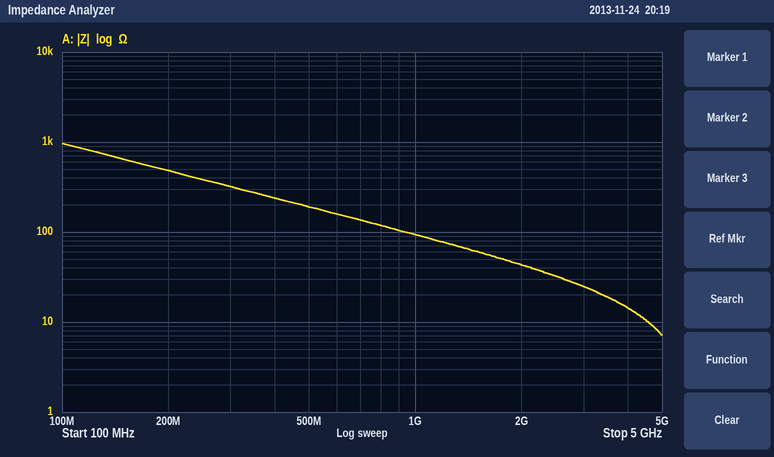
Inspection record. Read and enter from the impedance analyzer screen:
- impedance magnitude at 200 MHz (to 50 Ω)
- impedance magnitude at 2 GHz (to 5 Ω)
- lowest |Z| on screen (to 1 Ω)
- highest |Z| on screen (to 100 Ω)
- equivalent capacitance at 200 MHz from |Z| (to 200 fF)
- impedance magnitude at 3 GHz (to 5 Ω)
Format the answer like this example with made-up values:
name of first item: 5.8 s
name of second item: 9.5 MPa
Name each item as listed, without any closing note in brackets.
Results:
impedance magnitude at 200 MHz: 500 Ω
impedance magnitude at 2 GHz: 45 Ω
lowest |Z| on screen: 7 Ω
highest |Z| on screen: 1.0 kΩ
equivalent capacitance at 200 MHz from |Z|: 1.6 pF
impedance magnitude at 3 GHz: 25 Ω
